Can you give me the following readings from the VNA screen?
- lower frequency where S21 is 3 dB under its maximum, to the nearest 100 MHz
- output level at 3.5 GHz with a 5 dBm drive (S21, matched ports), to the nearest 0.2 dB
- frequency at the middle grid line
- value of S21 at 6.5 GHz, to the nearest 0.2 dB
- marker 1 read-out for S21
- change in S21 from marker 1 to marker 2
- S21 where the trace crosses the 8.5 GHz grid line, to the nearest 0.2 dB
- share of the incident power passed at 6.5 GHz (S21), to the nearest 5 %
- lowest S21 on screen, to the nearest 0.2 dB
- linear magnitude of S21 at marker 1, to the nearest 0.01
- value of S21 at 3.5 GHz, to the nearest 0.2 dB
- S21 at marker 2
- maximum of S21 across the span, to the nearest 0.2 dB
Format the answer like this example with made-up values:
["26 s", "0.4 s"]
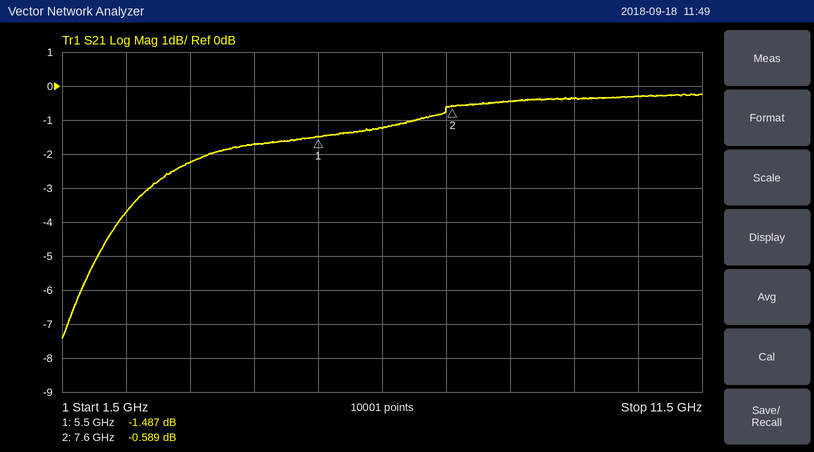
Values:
["2.7 GHz", "2.8 dBm", "6.5 GHz", "-1.2 dB", "-1.487 dB", "0.898 dB", "-0.4 dB", "75 %", "-7.4 dB", "0.84", "-2.2 dB", "-0.589 dB", "-0.2 dB"]
